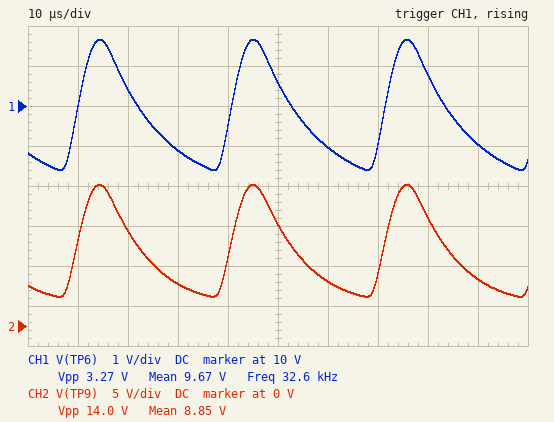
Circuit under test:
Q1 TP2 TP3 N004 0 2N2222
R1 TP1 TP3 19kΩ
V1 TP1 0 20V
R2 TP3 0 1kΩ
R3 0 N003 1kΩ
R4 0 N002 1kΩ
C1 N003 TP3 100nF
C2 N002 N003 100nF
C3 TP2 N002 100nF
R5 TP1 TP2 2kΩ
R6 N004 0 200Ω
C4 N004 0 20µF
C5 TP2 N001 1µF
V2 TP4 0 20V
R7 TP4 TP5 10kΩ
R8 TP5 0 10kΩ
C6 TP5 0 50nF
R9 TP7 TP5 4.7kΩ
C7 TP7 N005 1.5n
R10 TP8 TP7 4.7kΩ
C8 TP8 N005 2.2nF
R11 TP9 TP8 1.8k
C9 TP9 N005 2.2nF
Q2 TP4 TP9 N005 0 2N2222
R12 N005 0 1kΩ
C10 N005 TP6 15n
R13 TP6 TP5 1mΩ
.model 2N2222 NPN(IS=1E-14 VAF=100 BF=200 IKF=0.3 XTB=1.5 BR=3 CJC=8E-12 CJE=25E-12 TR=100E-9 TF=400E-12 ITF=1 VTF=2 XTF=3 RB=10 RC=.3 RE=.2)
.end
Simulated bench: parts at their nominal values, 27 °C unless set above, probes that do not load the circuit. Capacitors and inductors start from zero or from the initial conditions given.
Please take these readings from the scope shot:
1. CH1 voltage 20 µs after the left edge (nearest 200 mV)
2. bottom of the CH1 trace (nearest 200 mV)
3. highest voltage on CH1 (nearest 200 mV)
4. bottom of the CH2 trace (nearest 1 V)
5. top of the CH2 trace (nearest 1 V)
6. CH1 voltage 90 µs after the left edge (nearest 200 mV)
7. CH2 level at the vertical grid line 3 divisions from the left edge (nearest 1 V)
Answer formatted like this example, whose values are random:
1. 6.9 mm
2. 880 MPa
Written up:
1. 10.4 V
2. 8.4 V
3. 11.6 V
4. 4 V
5. 18 V
6. 9.0 V
7. 5 V
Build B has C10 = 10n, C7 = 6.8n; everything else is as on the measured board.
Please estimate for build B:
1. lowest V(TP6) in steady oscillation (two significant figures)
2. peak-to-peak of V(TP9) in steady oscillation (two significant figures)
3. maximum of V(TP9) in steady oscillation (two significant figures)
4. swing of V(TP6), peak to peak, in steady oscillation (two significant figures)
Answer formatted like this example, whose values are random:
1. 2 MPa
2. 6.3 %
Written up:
1. 8.6 V
2. 17 V
3. 19 V
4. 2.9 V
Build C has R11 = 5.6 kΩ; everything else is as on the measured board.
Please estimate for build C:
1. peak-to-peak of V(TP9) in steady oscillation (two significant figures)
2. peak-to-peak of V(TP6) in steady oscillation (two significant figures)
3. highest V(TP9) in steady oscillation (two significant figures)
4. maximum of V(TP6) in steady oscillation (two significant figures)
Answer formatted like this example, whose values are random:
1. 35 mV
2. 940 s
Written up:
1. 13 V
2. 3.0 V
3. 16 V
4. 11 V
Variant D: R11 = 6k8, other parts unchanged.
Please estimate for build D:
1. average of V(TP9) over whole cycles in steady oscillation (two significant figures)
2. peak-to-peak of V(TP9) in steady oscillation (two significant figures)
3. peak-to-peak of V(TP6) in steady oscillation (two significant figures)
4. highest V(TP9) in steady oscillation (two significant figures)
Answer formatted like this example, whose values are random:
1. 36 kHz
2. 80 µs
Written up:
1. 9.1 V
2. 11 V
3. 2.6 V
4. 15 V
